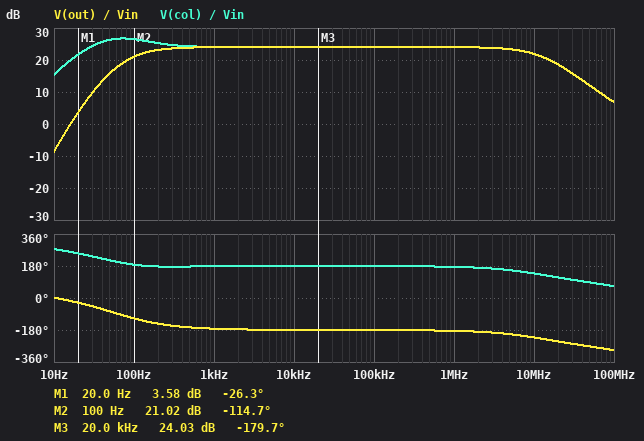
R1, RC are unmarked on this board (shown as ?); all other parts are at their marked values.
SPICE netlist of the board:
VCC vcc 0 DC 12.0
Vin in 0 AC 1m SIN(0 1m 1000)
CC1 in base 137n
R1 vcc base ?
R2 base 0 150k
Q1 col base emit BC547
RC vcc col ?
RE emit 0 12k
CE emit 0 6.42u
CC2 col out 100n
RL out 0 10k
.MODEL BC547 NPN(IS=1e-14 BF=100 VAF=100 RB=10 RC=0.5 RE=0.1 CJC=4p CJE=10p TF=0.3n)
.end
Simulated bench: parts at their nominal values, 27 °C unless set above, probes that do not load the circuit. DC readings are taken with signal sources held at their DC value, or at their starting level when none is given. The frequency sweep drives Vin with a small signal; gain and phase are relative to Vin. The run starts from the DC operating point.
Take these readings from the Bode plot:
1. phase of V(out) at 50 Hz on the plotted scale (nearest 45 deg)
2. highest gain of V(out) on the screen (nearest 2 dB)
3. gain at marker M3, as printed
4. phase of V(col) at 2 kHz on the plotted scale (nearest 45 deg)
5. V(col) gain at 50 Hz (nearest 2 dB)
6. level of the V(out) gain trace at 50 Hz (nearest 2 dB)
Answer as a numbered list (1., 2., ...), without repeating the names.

1. -90 deg
2. 24 dB
3. 24.03 dB
4. 180 deg
5. 26 dB
6. 16 dB
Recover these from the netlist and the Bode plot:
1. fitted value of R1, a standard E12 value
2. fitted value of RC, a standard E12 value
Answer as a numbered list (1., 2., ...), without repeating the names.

1. 1.2 MΩ
2. 27 kΩ
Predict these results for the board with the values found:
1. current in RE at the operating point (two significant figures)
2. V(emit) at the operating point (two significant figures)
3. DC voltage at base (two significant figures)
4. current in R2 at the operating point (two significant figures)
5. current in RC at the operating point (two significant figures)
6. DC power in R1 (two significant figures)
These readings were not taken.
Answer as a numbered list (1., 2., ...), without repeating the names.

1. 57 µA
2. 690 mV
3. 1.3 V
4. 8.4 µA
5. 57 µA
6. 96 µW
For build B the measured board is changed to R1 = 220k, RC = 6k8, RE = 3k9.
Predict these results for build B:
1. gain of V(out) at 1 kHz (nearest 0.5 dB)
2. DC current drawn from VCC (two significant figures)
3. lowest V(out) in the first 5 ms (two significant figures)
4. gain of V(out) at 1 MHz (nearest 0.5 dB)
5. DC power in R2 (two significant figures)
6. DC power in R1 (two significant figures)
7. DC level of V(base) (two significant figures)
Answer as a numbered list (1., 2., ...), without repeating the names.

1. 38.5 dB
2. 910 µA
3. -84 mV
4. 42.5 dB
5. 110 µW
6. 280 µW
7. 4.1 V
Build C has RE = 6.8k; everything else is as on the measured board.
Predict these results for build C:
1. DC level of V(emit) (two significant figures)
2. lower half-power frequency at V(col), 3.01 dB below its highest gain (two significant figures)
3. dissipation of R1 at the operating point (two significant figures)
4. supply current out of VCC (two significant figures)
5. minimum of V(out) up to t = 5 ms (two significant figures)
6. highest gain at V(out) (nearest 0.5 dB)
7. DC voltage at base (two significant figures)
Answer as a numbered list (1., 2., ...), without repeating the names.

1. 630 mV
2. 35 Hz
3. 97 µW
4. 100 µA
5. -26 mV
6. 28.0 dB
7. 1.2 V
